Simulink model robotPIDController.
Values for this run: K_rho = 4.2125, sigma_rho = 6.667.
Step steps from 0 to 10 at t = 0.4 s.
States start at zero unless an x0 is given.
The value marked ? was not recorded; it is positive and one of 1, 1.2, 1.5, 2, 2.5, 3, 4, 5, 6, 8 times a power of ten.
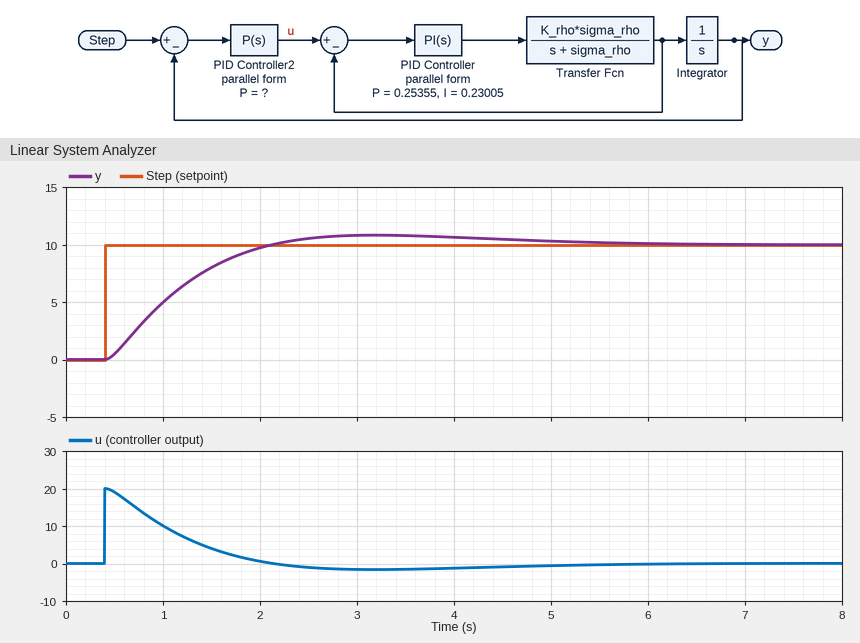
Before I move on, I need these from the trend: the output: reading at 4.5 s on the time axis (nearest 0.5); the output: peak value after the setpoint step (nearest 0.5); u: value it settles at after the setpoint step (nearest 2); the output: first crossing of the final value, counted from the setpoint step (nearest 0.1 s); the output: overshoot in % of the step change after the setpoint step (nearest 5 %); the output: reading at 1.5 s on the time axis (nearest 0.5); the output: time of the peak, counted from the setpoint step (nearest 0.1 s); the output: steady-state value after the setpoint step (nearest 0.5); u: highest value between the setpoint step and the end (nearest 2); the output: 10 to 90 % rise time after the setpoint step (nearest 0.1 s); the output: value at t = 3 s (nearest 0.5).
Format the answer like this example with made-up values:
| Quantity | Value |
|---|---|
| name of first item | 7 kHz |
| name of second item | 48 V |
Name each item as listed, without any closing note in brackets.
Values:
| Quantity | Value |
|---|---|
| the output: reading at 4.5 s on the time axis | 10.5 |
| the output: peak value after the setpoint step | 11.0 |
| u: value it settles at after the setpoint step | 0 |
| the output: first crossing of the final value, counted from the setpoint step | 1.7 s |
| the output: overshoot in % of the step change after the setpoint step | 10 % |
| the output: reading at 1.5 s on the time axis | 8.0 |
| the output: time of the peak, counted from the setpoint step | 2.8 s |
| the output: steady-state value after the setpoint step | 10.0 |
| u: highest value between the setpoint step and the end | 20 |
| the output: 10 to 90 % rise time after the setpoint step | 1.2 s |
| the output: value at t = 3 s | 11.0 |
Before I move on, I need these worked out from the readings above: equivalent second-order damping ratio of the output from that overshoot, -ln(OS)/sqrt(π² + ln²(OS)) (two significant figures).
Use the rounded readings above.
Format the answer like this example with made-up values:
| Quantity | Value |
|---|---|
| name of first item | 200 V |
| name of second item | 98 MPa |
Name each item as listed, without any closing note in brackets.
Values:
| Quantity | Value |
|---|---|
| equivalent second-order damping ratio of the output from that overshoot, -ln(OS)/sqrt(π² + ln²(OS)) | 0.59 |
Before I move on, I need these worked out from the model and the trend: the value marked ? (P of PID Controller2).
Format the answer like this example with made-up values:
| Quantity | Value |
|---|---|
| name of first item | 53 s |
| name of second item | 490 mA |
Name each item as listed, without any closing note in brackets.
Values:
| Quantity | Value |
|---|---|
| the value marked ? | 2 |
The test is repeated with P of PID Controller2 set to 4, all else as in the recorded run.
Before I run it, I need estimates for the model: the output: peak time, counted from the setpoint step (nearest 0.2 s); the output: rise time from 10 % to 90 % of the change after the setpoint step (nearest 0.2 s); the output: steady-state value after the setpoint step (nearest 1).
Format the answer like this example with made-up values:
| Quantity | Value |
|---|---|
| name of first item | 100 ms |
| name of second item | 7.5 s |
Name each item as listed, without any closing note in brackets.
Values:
| Quantity | Value |
|---|---|
| the output: peak time, counted from the setpoint step | 1.6 s |
| the output: rise time from 10 % to 90 % of the change after the setpoint step | 0.6 s |
| the output: steady-state value after the setpoint step | 10 |
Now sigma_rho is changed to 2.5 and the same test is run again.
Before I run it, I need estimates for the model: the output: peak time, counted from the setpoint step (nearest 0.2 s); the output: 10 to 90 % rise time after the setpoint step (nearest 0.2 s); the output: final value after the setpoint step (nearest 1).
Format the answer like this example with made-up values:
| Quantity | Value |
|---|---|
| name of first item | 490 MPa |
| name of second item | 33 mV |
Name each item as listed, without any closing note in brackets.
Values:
| Quantity | Value |
|---|---|
| the output: peak time, counted from the setpoint step | 2.4 s |
| the output: 10 to 90 % rise time after the setpoint step | 1.0 s |
| the output: final value after the setpoint step | 10 |
